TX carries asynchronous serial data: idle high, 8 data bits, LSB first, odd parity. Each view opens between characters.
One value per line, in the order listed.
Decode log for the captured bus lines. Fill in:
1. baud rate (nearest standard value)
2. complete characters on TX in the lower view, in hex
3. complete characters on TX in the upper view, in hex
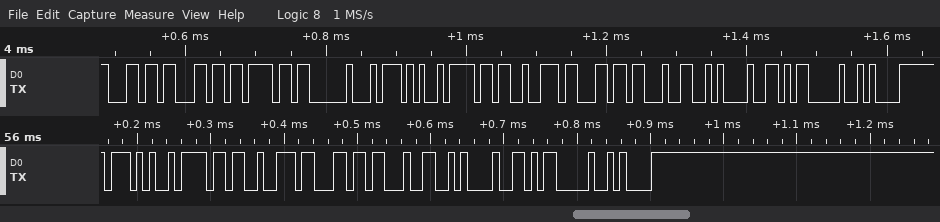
115200 baud
57, 6F, 72, 6C, 64, 21, 0D, 0A
6C, 6C, 6F, 20, 57, 6F, 72, 6C, 64, 21, 0D, 0A
